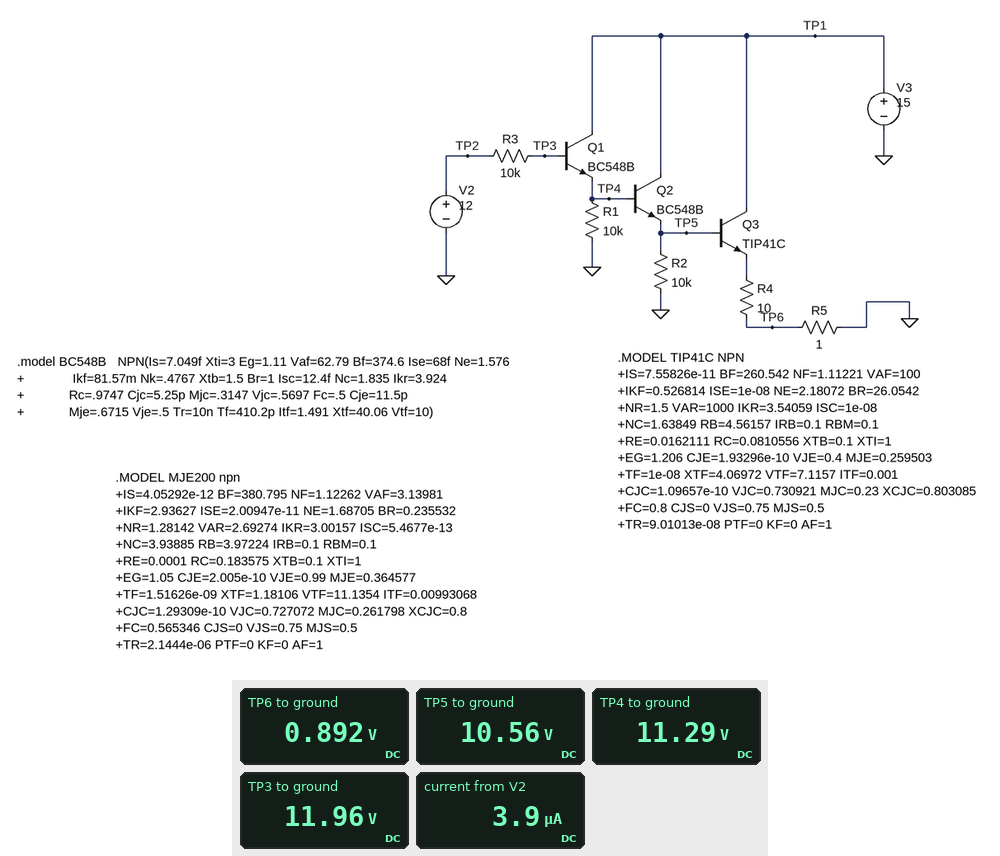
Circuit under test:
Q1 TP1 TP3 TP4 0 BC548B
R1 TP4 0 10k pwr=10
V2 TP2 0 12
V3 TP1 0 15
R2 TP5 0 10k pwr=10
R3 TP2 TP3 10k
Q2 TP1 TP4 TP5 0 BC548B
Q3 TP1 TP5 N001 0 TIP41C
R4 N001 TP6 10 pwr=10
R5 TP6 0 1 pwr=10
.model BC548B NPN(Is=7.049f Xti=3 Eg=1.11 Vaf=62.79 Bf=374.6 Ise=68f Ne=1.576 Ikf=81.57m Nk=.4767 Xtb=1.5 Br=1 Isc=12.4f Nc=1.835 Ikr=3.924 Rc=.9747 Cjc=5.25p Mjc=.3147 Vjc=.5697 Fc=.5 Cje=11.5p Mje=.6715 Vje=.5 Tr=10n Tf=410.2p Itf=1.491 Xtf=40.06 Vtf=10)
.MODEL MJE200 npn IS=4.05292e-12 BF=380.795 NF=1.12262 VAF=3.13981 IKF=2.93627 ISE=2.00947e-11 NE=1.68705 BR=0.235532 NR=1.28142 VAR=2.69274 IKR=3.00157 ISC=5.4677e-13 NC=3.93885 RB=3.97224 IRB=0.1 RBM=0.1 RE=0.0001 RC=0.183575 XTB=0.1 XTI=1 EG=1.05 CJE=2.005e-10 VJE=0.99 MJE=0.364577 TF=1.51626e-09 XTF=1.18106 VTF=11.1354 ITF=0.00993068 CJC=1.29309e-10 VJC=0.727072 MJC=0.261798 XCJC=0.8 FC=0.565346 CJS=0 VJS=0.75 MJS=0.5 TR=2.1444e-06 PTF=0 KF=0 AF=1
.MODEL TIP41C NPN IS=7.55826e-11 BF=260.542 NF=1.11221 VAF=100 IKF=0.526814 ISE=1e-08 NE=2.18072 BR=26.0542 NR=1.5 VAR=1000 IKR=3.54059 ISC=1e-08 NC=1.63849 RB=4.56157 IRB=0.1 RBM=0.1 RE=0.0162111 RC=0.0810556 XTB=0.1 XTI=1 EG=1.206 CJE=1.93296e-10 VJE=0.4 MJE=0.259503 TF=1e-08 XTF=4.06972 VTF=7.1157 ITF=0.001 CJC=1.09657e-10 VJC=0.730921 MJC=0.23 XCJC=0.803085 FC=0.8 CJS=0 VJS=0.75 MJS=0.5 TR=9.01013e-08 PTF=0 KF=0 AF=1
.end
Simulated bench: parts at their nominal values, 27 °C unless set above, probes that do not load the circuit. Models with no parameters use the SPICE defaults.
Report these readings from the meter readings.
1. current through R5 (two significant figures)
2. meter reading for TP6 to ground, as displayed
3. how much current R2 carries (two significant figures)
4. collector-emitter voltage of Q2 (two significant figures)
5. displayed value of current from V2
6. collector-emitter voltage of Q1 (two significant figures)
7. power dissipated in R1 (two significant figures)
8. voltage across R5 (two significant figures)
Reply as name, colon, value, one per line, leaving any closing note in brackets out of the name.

current through R5: 890 mA
meter reading for TP6 to ground, as displayed: 0.892 V
how much current R2 carries: 1.1 mA
collector-emitter voltage of Q2: 4.4 V
displayed value of current from V2: 3.9 µA
collector-emitter voltage of Q1: 3.7 V
power dissipated in R1: 13 mW
voltage across R5: 890 mV
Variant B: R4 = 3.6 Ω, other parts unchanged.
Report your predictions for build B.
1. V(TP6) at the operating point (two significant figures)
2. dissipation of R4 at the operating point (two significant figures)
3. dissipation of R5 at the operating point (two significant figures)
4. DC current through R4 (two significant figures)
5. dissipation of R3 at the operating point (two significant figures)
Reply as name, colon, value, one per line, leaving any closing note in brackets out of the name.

V(TP6) at the operating point: 2.1 V
dissipation of R4 at the operating point: 16 W
dissipation of R5 at the operating point: 4.4 W
DC current through R4: 2.1 A
dissipation of R3 at the operating point: 180 nW
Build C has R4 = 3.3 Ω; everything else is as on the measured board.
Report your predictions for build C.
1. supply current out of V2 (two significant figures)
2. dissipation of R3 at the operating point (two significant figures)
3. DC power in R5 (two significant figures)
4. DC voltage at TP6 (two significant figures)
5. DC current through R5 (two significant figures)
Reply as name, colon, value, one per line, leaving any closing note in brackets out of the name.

supply current out of V2: 4.3 µA
dissipation of R3 at the operating point: 190 nW
DC power in R5: 5.0 W
DC voltage at TP6: 2.2 V
DC current through R5: 2.2 A
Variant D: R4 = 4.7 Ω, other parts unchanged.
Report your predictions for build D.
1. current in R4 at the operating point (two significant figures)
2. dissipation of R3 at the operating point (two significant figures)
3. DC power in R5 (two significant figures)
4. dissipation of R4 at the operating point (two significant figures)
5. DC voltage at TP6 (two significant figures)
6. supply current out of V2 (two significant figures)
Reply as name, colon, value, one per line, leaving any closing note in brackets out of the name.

current in R4 at the operating point: 1.7 A
dissipation of R3 at the operating point: 170 nW
DC power in R5: 2.9 W
dissipation of R4 at the operating point: 14 W
DC voltage at TP6: 1.7 V
supply current out of V2: 4.1 µA
